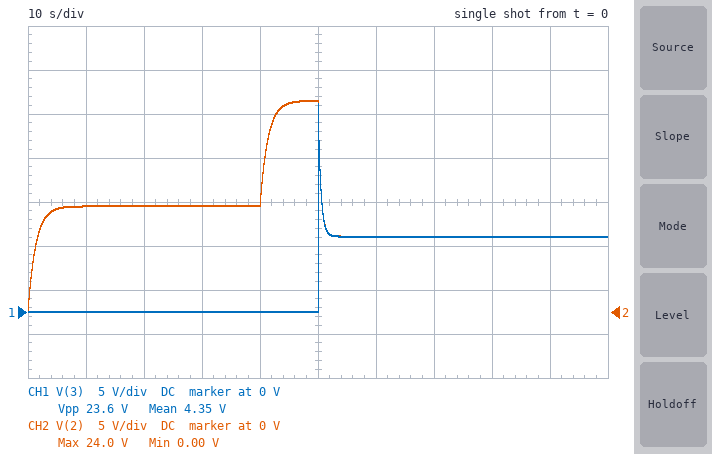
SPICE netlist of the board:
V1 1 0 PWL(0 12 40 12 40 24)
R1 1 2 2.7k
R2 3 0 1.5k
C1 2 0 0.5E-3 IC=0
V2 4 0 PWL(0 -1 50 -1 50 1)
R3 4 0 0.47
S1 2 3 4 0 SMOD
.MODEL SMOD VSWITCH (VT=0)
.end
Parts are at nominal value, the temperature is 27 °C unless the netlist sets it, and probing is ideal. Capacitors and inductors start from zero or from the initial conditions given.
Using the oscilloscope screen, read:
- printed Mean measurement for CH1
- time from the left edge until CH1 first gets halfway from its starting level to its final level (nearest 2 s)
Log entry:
4.35 V
50 s
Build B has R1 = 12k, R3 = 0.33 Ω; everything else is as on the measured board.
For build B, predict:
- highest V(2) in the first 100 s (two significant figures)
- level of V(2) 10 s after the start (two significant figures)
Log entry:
22 V
9.7 V
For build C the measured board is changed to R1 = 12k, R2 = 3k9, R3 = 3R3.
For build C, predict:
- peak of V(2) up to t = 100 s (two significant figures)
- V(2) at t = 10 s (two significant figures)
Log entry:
22 V
9.7 V
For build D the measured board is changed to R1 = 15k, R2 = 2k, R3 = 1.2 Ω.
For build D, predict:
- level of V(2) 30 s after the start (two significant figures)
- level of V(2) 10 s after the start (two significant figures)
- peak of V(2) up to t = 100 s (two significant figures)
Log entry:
12 V
8.8 V
21 V
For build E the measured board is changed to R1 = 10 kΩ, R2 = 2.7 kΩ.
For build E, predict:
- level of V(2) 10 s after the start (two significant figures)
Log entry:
10 V
